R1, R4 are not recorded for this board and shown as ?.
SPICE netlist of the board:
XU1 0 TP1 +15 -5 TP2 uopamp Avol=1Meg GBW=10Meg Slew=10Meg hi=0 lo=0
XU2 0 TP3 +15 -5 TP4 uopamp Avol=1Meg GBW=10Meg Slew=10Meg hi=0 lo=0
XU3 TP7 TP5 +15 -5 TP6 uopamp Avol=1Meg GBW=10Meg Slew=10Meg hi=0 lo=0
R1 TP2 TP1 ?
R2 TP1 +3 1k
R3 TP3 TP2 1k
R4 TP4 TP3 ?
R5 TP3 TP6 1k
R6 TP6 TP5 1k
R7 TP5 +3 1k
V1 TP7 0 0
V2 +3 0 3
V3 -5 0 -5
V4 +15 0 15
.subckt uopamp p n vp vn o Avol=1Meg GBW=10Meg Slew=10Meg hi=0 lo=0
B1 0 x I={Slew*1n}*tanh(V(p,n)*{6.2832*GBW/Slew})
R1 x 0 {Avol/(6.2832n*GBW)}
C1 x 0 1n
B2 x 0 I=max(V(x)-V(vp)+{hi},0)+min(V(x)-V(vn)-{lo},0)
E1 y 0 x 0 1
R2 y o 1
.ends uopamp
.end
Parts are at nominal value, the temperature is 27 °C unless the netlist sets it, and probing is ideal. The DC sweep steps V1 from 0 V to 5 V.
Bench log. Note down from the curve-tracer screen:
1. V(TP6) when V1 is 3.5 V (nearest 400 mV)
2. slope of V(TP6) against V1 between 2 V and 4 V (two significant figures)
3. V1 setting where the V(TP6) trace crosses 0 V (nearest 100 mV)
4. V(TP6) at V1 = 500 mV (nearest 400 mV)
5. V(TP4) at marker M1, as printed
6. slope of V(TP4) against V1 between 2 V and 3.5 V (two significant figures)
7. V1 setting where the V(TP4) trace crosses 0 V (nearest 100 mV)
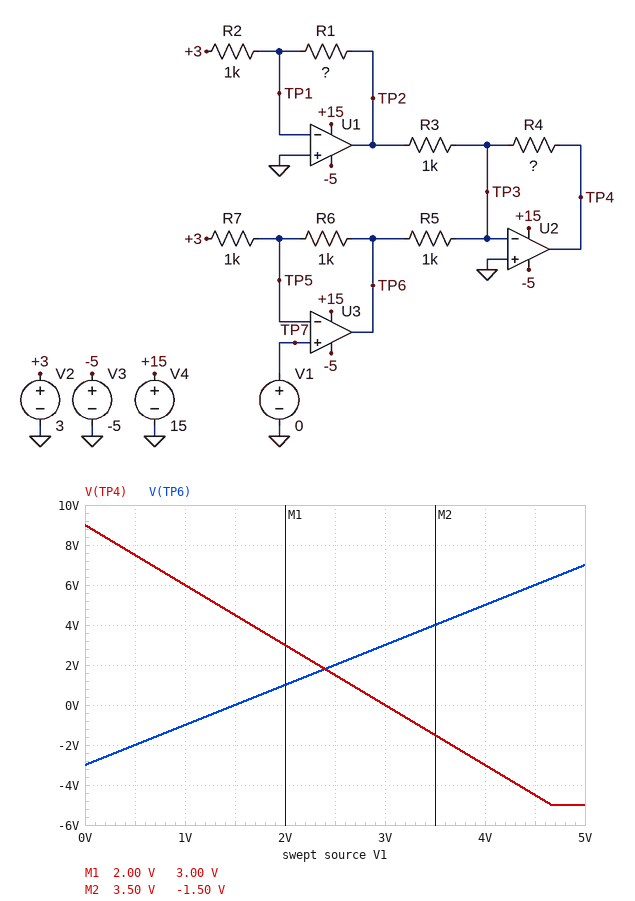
4.0 V
2.0 V/V
1.5 V
-2.0 V
3.00 V
-3.0 V/V
3.0 V
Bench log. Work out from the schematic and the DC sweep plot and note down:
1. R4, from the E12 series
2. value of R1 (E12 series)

1.5 kΩ
1 kΩ
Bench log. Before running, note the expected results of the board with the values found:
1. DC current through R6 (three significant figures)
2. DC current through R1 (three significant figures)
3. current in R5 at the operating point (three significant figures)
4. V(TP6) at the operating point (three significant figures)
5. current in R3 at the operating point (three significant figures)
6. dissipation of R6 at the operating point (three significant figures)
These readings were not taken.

3.00 mA
3.00 mA
3.00 mA
-3.00 V
3.00 mA
9.00 mW
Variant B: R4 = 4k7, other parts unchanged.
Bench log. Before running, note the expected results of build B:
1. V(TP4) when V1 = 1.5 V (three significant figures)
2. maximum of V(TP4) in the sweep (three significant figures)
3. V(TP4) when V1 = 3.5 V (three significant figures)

14.1 V
15.0 V
-4.70 V
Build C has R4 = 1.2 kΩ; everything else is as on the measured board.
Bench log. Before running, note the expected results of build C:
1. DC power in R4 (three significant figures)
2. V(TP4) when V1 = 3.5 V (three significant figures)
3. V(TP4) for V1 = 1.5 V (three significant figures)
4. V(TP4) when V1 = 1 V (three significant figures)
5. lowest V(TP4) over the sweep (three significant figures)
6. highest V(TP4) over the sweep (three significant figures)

43.2 mW
-1.20 V
3.60 V
4.80 V
-4.80 V
7.20 V
